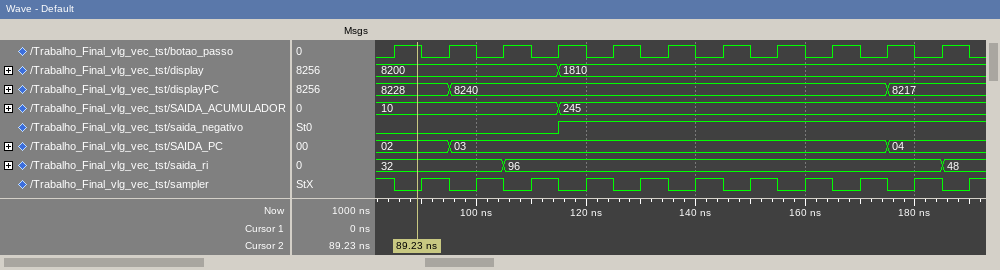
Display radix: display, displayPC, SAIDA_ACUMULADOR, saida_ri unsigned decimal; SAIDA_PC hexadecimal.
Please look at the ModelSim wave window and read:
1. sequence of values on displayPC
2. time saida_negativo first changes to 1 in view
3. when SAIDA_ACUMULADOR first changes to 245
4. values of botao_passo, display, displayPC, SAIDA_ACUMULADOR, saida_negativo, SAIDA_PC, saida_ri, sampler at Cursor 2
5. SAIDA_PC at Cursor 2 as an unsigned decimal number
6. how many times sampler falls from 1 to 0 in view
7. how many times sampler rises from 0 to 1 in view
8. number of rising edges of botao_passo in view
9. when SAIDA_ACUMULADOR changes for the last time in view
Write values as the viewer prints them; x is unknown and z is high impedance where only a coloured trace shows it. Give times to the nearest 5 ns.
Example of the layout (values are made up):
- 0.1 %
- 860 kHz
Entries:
- 8228, 8240, 8217
- 115 ns
- 115 ns
- botao_passo=1, display=8200, displayPC=8228, SAIDA_ACUMULADOR=10, saida_negativo=0, SAIDA_PC=02, saida_ri=32, sampler=0
- 2
- 11
- 11
- 11
- 115 ns
